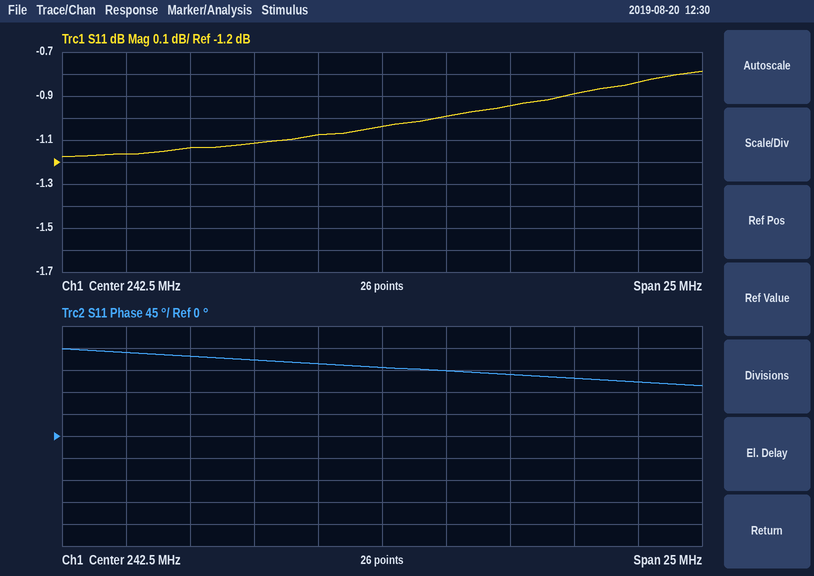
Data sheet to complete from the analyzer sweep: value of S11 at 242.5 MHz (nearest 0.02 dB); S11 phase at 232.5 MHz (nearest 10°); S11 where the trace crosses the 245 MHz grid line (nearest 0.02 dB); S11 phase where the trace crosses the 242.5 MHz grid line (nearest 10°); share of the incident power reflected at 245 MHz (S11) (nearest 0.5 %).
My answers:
-1.04 dB
170°
-1.00 dB
140°
79.5 %
